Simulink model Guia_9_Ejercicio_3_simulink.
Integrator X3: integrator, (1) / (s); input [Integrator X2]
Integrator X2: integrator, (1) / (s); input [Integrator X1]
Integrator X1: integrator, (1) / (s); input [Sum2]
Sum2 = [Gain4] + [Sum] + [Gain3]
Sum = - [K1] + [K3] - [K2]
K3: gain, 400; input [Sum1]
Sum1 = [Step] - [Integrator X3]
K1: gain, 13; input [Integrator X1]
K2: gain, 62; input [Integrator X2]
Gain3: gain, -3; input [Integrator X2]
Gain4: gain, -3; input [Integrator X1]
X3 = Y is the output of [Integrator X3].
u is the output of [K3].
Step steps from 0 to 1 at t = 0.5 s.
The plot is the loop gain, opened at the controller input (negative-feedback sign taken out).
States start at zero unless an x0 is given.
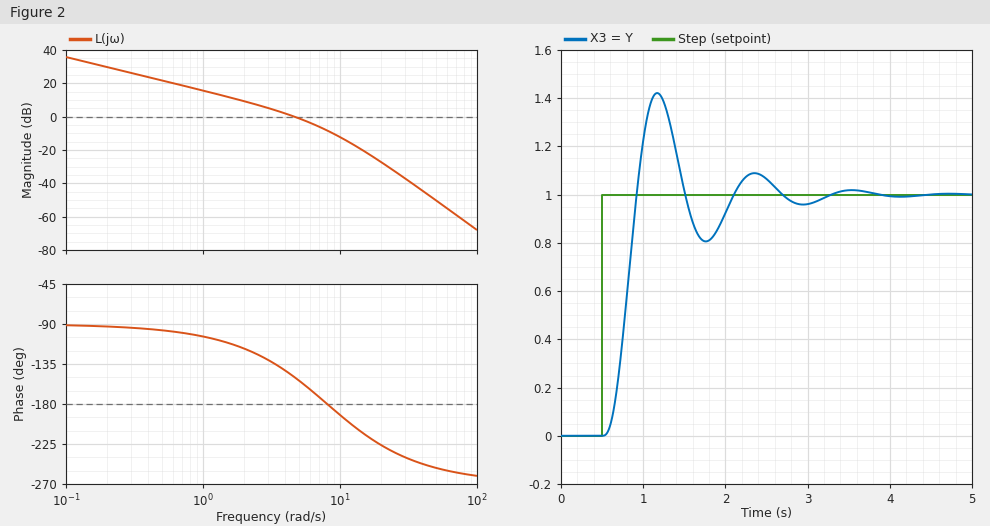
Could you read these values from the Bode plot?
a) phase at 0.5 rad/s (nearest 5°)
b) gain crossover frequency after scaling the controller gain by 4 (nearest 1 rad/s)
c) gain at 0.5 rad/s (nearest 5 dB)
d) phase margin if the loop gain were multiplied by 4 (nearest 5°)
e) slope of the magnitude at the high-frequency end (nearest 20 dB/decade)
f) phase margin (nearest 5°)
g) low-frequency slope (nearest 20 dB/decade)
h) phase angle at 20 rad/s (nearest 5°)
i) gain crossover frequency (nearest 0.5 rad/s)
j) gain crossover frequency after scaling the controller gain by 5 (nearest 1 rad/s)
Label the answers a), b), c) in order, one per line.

a) -95°
b) 10 rad/s
c) 20 dB
d) -10°
e) -60 dB/decade
f) 30°
g) -20 dB/decade
h) -225°
i) 4.5 rad/s
j) 11 rad/s
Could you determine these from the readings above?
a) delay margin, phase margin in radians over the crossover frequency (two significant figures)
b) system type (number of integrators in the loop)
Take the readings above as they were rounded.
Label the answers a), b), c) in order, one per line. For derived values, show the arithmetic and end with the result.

a) 30 × π / 180 / 4.5 = 0.12 s
b) 1
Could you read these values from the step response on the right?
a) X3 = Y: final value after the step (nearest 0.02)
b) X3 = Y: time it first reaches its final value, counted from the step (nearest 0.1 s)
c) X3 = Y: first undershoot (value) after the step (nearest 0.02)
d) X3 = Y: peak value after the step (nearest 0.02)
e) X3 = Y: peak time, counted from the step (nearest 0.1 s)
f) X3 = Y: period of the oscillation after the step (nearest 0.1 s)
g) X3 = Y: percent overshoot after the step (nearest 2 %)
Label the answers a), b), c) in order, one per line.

a) 1.00
b) 0.4 s
c) 0.80
d) 1.42
e) 0.7 s
f) 1.2 s
g) 42 %
